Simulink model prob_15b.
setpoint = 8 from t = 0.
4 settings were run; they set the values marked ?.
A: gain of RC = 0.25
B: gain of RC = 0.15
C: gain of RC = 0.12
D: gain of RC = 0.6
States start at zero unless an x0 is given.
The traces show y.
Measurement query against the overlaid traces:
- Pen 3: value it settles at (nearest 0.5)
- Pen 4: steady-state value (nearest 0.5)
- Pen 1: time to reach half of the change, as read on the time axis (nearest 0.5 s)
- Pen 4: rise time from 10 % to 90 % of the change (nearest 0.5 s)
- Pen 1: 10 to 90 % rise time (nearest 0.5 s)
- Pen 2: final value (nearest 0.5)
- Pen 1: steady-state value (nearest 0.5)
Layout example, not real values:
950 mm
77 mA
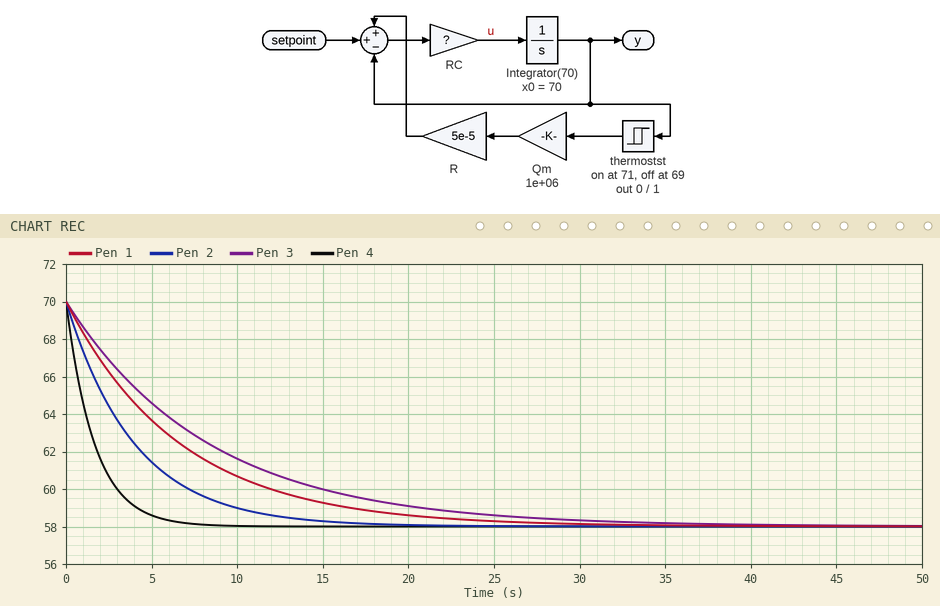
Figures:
58.0
58.0
4.5 s
3.5 s
14.5 s
58.0
58.0
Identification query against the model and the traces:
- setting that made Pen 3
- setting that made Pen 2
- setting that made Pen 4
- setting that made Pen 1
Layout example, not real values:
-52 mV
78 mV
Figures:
C
A
D
B
